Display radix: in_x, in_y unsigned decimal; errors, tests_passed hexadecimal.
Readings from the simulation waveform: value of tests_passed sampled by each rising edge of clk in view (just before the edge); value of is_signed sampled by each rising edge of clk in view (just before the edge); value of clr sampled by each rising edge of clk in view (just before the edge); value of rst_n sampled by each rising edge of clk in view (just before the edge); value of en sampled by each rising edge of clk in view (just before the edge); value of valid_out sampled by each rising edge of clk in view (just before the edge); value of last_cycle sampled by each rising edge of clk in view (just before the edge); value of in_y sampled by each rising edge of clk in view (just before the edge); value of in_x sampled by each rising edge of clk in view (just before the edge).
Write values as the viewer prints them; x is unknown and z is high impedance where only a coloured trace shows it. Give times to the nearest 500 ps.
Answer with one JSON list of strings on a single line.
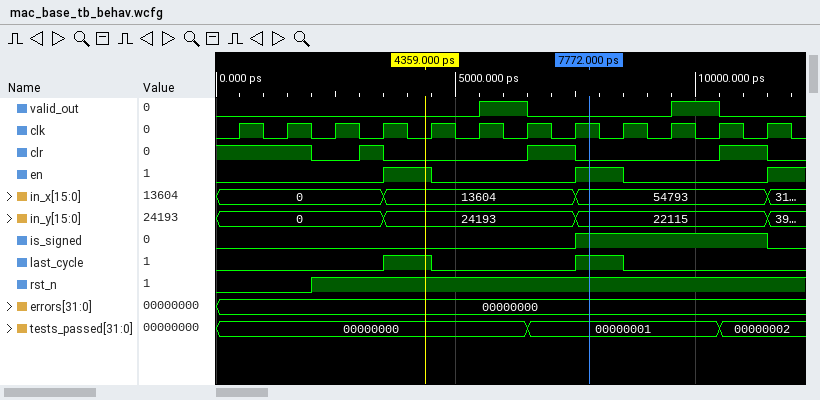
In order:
["00000000, 00000000, 00000000, 00000000, 00000000, 00000000, 00000000, 00000001, 00000001, 00000001, 00000001, 00000002", "0 0 0 0 0 0 0 0 1 1 1 1", "1 1 0 1 0 0 0 1 0 0 0 1", "0 0 1 1 1 1 1 1 1 1 1 1", "0 0 0 0 1 0 0 0 1 0 0 0", "0 0 0 0 0 0 1 0 0 0 1 0", "0 0 0 0 1 0 0 0 1 0 0 0", "0, 0, 0, 0, 24193, 24193, 24193, 24193, 22115, 22115, 22115, 22115", "0, 0, 0, 0, 13604, 13604, 13604, 13604, 54793, 54793, 54793, 54793"]
